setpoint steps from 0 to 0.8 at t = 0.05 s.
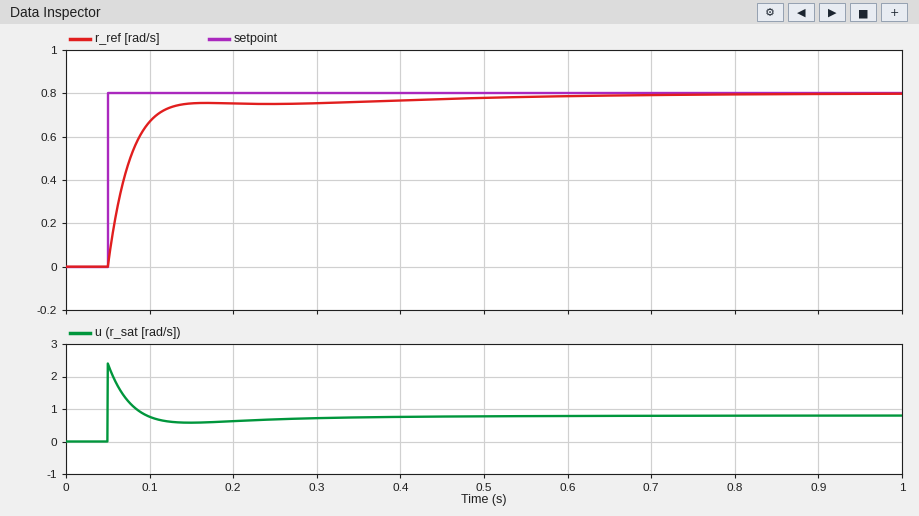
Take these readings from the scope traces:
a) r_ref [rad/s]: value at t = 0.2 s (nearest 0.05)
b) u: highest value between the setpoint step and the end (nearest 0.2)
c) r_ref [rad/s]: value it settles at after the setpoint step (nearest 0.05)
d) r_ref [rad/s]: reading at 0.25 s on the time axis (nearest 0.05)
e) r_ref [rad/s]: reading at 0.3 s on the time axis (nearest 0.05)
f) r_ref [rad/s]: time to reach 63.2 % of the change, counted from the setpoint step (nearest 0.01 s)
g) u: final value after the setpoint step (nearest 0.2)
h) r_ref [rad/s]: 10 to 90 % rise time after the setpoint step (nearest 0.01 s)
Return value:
0.75
2.4
0.80
0.75
0.75
0.03 s
0.8
0.06 s
